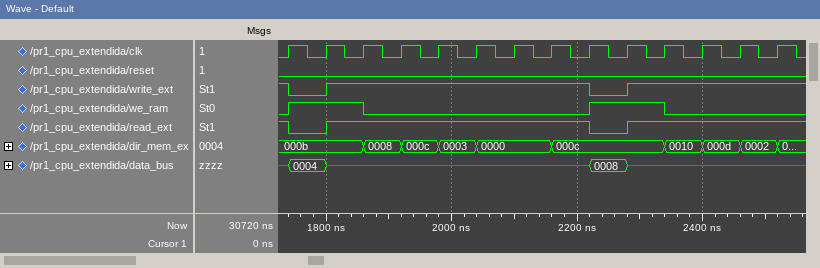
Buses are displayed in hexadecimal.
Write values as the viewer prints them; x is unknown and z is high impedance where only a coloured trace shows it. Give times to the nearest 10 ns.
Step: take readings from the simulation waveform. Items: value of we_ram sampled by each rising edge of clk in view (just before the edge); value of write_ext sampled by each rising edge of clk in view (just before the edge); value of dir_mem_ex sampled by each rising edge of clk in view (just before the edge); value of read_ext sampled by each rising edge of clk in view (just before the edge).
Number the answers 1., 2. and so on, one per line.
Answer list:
1. 0 1 1 0 0 0 0 0 0 1 1 0 0 0
2. 1 0 1 1 1 1 1 1 1 0 1 1 1 1
3. 000b, 000b, 000b, 0008, 000c, 0003, 0000, 0000, 000c, 000c, 000c, 0010, 000d, 0002
4. 1 0 1 1 1 1 1 1 1 0 1 1 1 1
